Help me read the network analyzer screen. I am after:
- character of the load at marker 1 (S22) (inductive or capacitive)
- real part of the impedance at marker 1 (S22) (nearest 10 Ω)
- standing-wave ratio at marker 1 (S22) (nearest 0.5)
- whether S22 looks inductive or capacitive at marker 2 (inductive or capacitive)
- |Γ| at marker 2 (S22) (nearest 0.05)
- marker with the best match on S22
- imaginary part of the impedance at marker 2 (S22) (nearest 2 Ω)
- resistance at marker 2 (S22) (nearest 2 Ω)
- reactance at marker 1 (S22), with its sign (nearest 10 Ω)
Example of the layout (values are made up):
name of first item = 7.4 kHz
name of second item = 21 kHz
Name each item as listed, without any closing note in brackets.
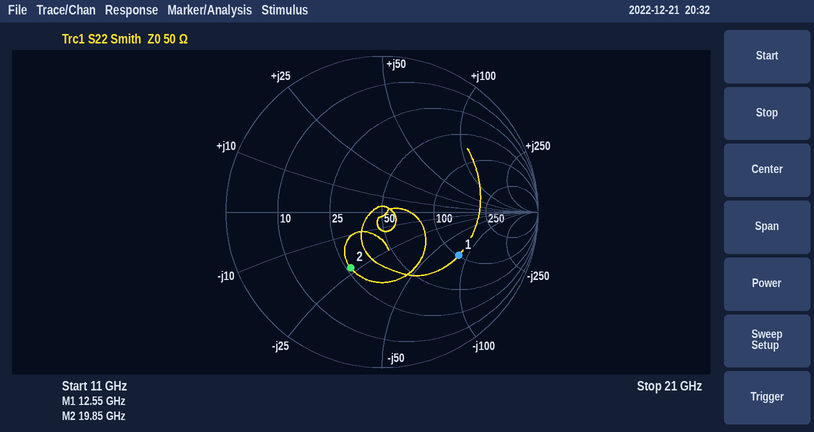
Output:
character of the load at marker 1 (S22) = capacitive
real part of the impedance at marker 1 (S22) = 100 Ω
standing-wave ratio at marker 1 (S22) = 3.5
whether S22 looks inductive or capacitive at marker 2 = capacitive
|Γ| at marker 2 (S22) = 0.40
marker with the best match on S22 = marker 2
imaginary part of the impedance at marker 2 (S22) = -22 Ω
resistance at marker 2 (S22) = 26 Ω
reactance at marker 1 (S22), with its sign = -80 Ω
